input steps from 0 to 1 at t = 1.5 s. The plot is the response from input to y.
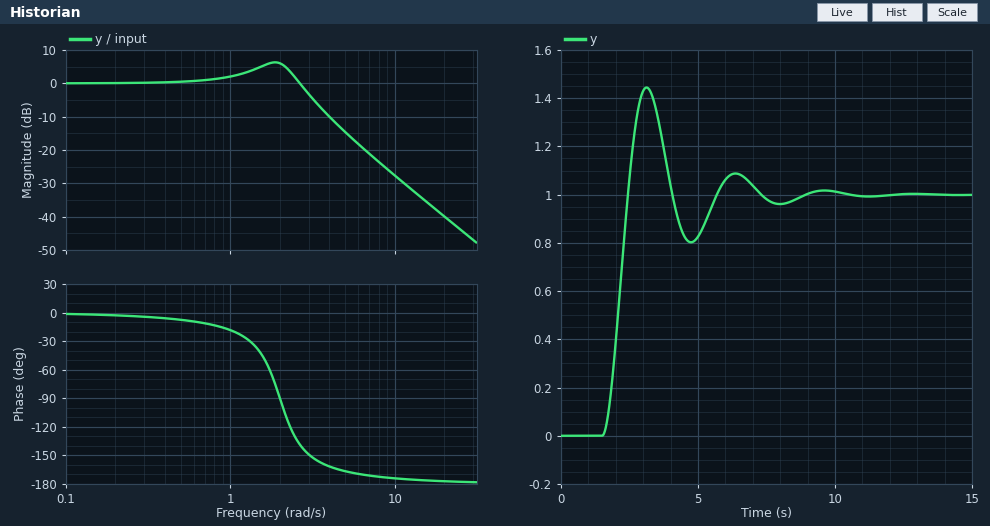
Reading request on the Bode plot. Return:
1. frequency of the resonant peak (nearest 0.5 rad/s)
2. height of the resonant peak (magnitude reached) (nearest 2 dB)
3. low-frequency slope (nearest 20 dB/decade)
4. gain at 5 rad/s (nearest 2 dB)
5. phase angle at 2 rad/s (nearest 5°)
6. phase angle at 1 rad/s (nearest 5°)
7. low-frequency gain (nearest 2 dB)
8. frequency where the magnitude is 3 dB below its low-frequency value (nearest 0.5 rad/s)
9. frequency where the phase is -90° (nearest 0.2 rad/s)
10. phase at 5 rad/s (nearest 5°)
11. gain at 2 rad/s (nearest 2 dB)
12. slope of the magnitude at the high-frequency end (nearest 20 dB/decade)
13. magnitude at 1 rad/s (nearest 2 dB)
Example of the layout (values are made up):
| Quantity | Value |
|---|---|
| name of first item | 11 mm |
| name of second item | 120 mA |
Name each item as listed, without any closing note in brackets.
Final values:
| Quantity | Value |
|---|---|
| frequency of the resonant peak | 2.0 rad/s |
| height of the resonant peak (magnitude reached) | 6 dB |
| low-frequency slope | 0 dB/decade |
| gain at 5 rad/s | -14 dB |
| phase angle at 2 rad/s | -90° |
| phase angle at 1 rad/s | -20° |
| low-frequency gain | 0 dB |
| frequency where the magnitude is 3 dB below its low-frequency value | 3.0 rad/s |
| frequency where the phase is -90° | 2.0 rad/s |
| phase at 5 rad/s | -165° |
| gain at 2 rad/s | 6 dB |
| slope of the magnitude at the high-frequency end | -40 dB/decade |
| magnitude at 1 rad/s | 2 dB |
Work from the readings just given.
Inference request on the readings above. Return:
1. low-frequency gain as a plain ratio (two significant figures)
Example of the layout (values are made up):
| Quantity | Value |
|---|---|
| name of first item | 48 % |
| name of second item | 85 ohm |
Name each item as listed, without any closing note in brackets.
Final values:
| Quantity | Value |
|---|---|
| low-frequency gain as a plain ratio | 1.0 |
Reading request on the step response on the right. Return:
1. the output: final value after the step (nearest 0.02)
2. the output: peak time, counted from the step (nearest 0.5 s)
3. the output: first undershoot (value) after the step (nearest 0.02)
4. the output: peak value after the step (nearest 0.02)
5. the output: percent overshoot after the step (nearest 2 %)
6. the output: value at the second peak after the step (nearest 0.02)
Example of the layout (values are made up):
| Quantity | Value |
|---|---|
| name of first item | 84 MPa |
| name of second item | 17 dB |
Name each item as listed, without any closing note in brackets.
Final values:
| Quantity | Value |
|---|---|
| the output: final value after the step | 1.00 |
| the output: peak time, counted from the step | 1.5 s |
| the output: first undershoot (value) after the step | 0.80 |
| the output: peak value after the step | 1.44 |
| the output: percent overshoot after the step | 44 % |
| the output: value at the second peak after the step | 1.08 |
